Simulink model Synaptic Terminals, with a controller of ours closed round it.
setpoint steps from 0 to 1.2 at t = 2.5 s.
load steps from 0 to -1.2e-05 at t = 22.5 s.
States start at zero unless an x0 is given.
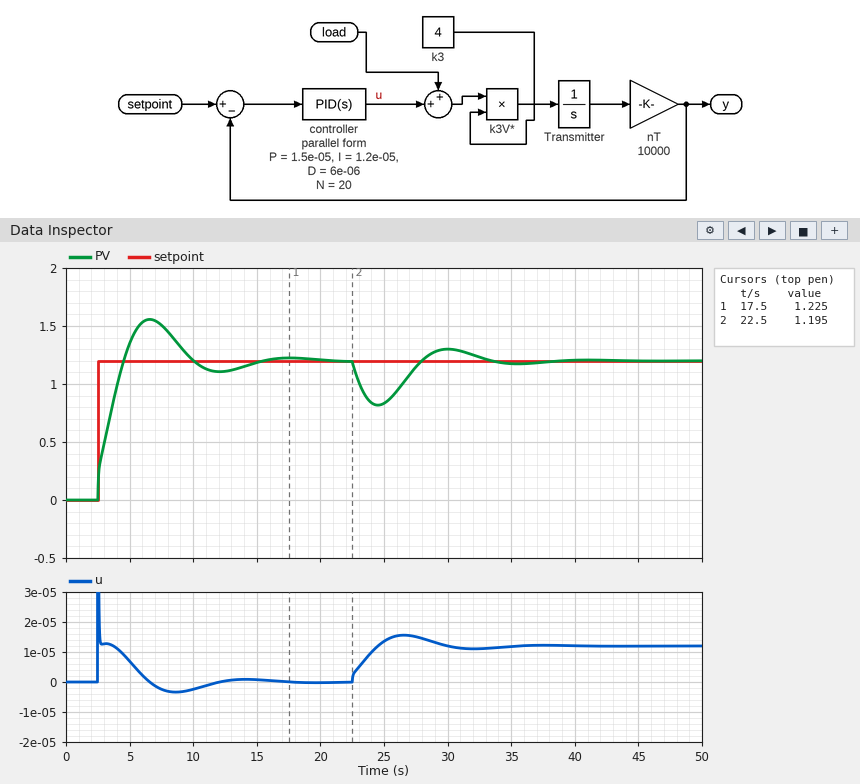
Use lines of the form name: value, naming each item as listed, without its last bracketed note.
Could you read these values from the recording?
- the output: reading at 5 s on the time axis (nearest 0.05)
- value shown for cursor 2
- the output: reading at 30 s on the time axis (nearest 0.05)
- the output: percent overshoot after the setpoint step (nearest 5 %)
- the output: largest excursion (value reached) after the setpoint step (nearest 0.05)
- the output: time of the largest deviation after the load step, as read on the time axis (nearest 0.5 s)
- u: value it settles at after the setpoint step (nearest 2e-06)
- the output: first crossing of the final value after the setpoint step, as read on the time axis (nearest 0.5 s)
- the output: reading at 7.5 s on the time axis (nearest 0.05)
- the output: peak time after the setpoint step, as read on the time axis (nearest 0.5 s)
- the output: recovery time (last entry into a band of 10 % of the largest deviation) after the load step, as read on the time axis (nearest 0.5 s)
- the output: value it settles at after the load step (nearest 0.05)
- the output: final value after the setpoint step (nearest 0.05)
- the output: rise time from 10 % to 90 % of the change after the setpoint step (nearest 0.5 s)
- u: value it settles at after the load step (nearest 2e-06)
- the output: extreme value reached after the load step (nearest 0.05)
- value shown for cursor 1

the output: reading at 5 s on the time axis: 1.35
value shown for cursor 2: 1.195
the output: reading at 30 s on the time axis: 1.30
the output: percent overshoot after the setpoint step: 30 %
the output: largest excursion (value reached) after the setpoint step: 1.55
the output: time of the largest deviation after the load step, as read on the time axis: 24.5 s
u: value it settles at after the setpoint step: 0.000000
the output: first crossing of the final value after the setpoint step, as read on the time axis: 4.5 s
the output: reading at 7.5 s on the time axis: 1.50
the output: peak time after the setpoint step, as read on the time axis: 6.5 s
the output: recovery time (last entry into a band of 10 % of the largest deviation) after the load step, as read on the time axis: 32.5 s
the output: value it settles at after the load step: 1.20
the output: final value after the setpoint step: 1.20
the output: rise time from 10 % to 90 % of the change after the setpoint step: 1.5 s
u: value it settles at after the load step: 0.000012
the output: extreme value reached after the load step: 0.80
value shown for cursor 1: 1.225
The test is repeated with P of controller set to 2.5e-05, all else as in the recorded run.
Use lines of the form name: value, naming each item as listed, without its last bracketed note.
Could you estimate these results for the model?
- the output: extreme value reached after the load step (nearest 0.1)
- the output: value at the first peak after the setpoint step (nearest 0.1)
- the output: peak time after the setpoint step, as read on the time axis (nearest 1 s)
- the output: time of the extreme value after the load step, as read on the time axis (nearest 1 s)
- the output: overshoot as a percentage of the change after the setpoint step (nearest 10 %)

the output: extreme value reached after the load step: 0.9
the output: value at the first peak after the setpoint step: 1.4
the output: peak time after the setpoint step, as read on the time axis: 6 s
the output: time of the extreme value after the load step, as read on the time axis: 24 s
the output: overshoot as a percentage of the change after the setpoint step: 20 %
